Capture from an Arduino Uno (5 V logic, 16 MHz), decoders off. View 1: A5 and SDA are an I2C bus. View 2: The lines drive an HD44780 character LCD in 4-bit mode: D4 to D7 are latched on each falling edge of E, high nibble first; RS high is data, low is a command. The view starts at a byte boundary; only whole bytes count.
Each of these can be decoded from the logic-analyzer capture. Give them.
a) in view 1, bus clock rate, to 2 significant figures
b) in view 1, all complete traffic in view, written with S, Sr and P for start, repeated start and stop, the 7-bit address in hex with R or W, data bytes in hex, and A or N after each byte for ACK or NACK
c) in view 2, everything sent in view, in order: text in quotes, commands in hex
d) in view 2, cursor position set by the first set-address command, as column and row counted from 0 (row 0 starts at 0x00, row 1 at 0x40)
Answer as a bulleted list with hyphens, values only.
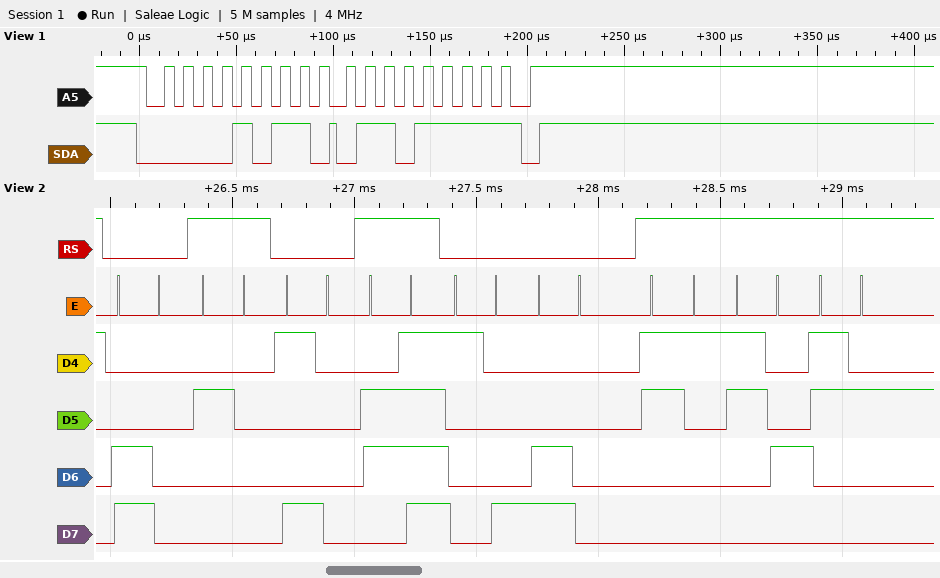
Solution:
- 100 kHz
- S 05R A 6F N P
- 0xC0 " " 0x90 "o" 0x18 0xC0 "142"
- column 0, row 1
